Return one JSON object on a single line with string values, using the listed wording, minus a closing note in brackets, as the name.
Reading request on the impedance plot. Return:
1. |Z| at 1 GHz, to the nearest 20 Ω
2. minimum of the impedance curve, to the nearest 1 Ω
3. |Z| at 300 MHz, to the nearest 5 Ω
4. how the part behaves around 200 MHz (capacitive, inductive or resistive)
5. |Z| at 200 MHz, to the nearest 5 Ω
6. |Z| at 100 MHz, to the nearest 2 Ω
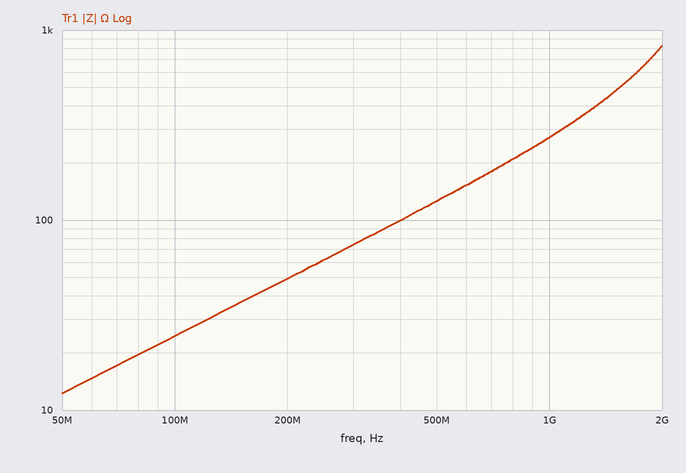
{"|Z| at 1 GHz, to the nearest 20 Ω": "280 Ω", "minimum of the impedance curve, to the nearest 1 Ω": "12 Ω", "|Z| at 300 MHz, to the nearest 5 Ω": "75 Ω", "how the part behaves around 200 MHz": "inductive", "|Z| at 200 MHz, to the nearest 5 Ω": "50 Ω", "|Z| at 100 MHz, to the nearest 2 Ω": "24 Ω"}
